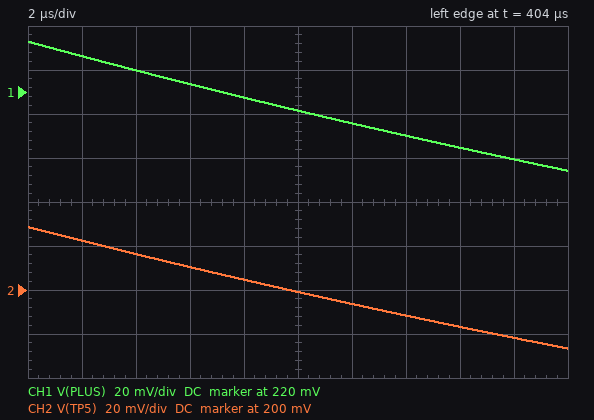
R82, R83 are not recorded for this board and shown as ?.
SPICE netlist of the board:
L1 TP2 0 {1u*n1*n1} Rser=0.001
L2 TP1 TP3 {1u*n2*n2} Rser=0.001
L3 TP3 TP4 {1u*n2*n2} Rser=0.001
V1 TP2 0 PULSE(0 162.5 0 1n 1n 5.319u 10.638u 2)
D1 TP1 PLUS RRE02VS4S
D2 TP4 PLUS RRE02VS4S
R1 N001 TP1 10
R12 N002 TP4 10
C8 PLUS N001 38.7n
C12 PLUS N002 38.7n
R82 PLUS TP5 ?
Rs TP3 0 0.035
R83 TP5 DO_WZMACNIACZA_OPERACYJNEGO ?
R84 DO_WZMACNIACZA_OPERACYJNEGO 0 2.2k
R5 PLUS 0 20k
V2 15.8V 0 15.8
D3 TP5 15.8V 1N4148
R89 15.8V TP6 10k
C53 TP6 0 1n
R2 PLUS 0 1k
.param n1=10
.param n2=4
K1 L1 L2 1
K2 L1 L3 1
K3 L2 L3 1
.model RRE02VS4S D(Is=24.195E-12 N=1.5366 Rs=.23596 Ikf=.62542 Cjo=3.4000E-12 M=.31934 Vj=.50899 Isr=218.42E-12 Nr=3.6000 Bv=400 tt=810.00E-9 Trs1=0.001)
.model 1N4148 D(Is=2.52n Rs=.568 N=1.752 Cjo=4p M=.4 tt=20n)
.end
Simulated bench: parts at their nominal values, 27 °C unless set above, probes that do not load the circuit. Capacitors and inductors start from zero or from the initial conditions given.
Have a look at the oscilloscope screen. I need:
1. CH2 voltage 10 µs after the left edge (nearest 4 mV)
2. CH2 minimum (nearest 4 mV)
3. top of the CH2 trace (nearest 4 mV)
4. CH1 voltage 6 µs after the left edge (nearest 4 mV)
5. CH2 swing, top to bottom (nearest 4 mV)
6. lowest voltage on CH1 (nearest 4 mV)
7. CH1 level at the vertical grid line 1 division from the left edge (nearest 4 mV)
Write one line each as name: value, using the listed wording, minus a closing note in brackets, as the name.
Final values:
CH2 voltage 10 µs after the left edge: 200 mV
CH2 minimum: 172 mV
top of the CH2 trace: 228 mV
CH1 voltage 6 µs after the left edge: 224 mV
CH2 swing, top to bottom: 56 mV
lowest voltage on CH1: 184 mV
CH1 level at the vertical grid line 1 division from the left edge: 236 mV
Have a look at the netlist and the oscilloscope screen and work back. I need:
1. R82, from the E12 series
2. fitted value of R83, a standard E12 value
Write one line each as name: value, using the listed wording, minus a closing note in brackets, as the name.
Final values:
R82, from the E12 series: 2.2 kΩ
fitted value of R83, a standard E12 value: 33 kΩ
